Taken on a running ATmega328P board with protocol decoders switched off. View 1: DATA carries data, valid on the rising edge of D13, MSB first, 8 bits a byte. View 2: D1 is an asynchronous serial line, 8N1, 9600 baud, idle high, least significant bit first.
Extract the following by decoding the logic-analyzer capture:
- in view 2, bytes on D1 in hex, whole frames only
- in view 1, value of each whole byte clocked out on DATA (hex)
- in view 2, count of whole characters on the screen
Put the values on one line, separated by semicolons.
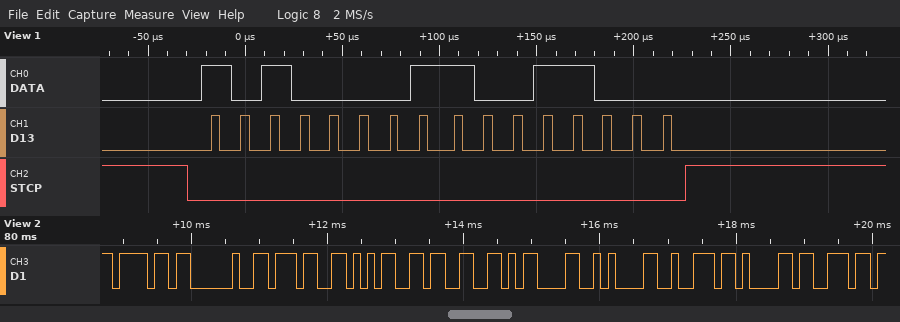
0x6F 0x20 0x37 0x35 0x33 0x0D 0x0A 0x72 0x61 0x6E; A1 98; 10
